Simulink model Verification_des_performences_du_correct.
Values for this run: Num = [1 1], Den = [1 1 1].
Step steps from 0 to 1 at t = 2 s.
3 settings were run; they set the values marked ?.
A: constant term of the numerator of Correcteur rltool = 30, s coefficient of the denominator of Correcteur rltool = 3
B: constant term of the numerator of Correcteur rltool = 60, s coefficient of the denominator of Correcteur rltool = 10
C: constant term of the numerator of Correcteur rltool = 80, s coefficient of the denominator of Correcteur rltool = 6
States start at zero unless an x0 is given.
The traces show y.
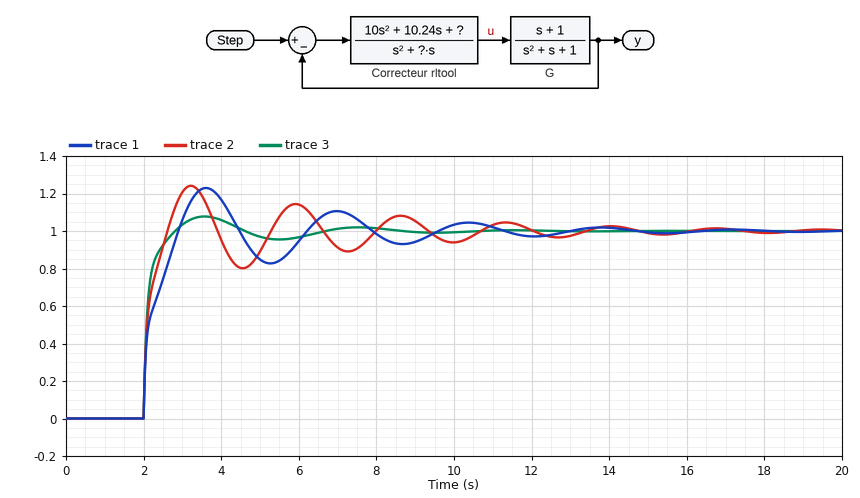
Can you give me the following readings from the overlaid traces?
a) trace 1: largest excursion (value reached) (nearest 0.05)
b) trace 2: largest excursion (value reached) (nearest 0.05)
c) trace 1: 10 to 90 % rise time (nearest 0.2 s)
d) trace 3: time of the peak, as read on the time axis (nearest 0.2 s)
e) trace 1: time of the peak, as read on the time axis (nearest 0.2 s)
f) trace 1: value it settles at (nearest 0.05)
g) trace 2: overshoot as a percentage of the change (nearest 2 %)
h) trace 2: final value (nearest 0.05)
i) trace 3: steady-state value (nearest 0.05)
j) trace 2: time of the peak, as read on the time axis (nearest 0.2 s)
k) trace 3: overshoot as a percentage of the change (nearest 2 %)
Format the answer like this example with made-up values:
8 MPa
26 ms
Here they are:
1.25
1.25
0.8 s
3.6 s
3.6 s
1.00
24 %
1.00
1.00
3.2 s
8 %
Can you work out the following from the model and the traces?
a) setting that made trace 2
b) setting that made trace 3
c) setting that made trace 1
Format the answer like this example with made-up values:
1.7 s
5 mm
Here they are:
C
A
B
